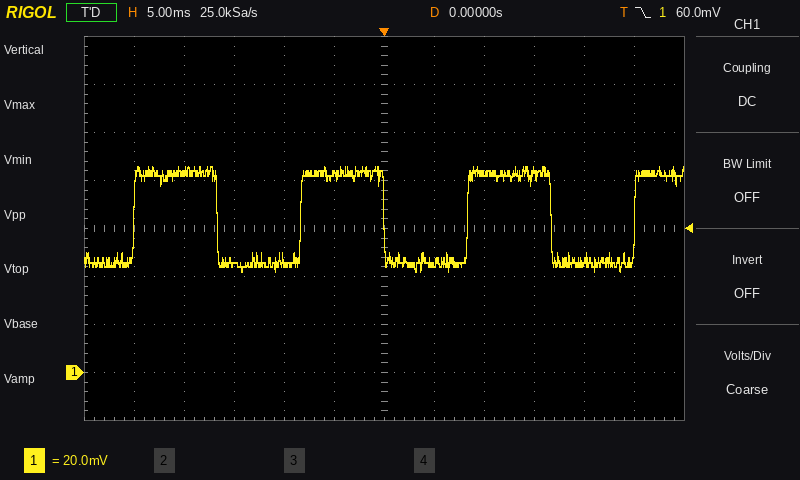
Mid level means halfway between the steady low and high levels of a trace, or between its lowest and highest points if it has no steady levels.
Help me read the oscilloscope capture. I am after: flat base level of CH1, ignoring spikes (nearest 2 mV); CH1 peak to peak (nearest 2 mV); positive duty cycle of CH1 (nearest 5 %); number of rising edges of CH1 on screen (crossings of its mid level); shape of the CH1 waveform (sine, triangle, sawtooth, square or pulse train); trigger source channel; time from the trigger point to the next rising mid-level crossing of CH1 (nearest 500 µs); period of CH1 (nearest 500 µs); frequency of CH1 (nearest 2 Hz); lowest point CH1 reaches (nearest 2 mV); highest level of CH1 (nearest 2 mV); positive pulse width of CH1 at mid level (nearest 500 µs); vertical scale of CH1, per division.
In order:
46 mV
44 mV
50 %
4
square
CH1
8.5 ms
16.5 ms
60 Hz
42 mV
86 mV
8.5 ms
20 mV
